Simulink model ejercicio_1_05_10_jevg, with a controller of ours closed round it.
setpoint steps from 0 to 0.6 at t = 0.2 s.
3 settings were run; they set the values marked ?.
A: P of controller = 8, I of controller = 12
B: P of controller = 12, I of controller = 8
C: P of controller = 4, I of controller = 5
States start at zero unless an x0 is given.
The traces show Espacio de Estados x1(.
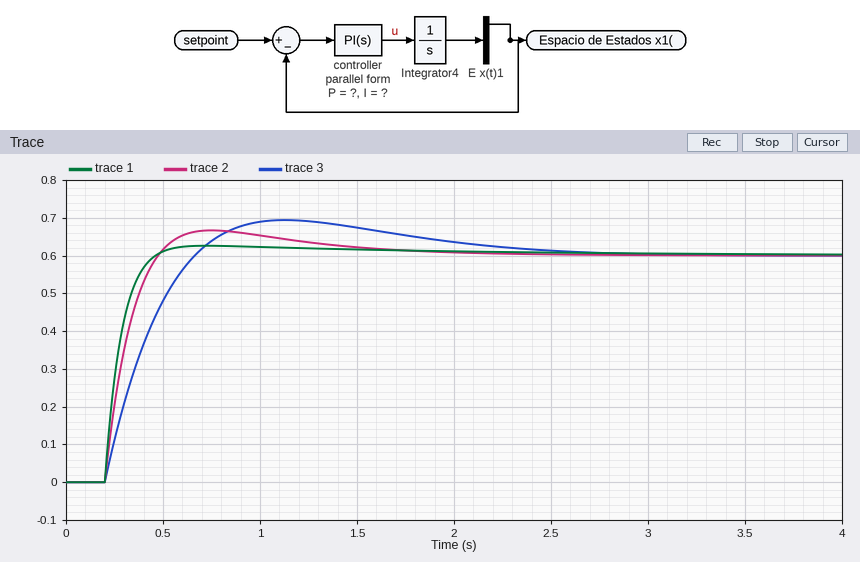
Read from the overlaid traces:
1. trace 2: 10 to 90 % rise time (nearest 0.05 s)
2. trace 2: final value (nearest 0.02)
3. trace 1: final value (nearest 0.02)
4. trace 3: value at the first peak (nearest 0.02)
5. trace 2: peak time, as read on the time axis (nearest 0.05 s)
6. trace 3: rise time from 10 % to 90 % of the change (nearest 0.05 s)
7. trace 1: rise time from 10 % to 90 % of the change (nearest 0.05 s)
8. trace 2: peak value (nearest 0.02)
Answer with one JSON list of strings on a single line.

["0.20 s", "0.60", "0.60", "0.70", "0.75 s", "0.35 s", "0.15 s", "0.66"]
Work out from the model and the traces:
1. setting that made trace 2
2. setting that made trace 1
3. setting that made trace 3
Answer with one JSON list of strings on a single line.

["A", "B", "C"]
